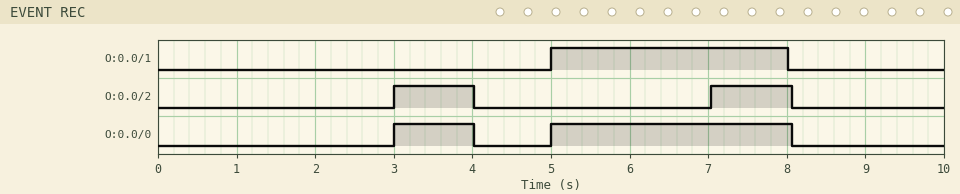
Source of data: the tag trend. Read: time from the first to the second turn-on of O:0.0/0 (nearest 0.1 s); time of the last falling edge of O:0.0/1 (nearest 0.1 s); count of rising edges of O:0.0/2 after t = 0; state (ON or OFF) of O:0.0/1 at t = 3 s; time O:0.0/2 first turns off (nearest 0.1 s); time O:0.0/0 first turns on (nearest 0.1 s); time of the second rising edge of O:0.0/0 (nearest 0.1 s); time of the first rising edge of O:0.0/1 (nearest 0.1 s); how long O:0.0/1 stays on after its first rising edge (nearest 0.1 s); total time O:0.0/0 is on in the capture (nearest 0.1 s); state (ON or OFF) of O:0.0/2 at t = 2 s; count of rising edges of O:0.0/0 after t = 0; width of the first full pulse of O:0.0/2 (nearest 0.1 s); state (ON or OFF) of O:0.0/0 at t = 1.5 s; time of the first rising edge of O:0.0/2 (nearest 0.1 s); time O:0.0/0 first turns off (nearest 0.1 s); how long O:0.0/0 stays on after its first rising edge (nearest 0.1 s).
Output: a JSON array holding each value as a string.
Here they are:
["2.0 s", "8.0 s", "2", "OFF", "4.0 s", "3.0 s", "5.0 s", "5.0 s", "3.0 s", "4.1 s", "OFF", "2", "1.0 s", "OFF", "3.0 s", "4.0 s", "1.0 s"]
